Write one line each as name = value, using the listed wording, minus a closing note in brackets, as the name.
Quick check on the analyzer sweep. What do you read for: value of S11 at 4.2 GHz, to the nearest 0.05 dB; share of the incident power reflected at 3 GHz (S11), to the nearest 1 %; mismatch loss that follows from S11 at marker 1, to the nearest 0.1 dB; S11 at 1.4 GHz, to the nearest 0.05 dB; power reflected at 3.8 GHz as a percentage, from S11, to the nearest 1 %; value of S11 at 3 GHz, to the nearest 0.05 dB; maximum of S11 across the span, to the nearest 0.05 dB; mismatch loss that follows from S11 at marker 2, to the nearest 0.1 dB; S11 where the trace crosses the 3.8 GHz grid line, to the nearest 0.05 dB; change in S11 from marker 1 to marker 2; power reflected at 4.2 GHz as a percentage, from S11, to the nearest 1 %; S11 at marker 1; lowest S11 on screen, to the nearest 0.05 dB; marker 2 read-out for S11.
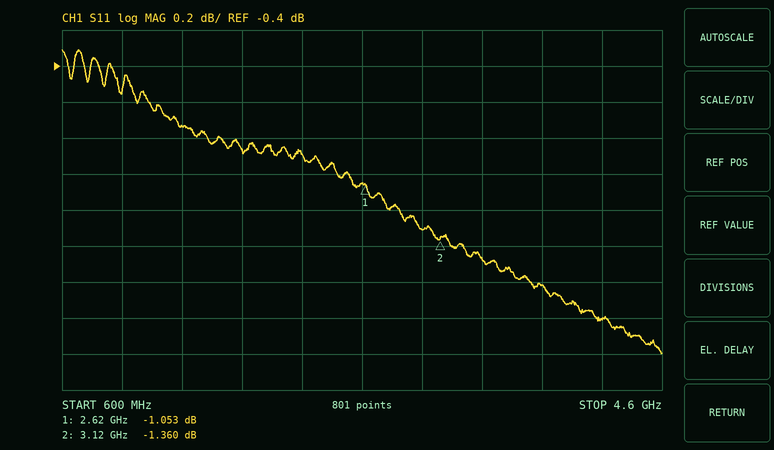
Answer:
value of S11 at 4.2 GHz, to the nearest 0.05 dB = -1.80 dB
share of the incident power reflected at 3 GHz (S11), to the nearest 1 % = 74 %
mismatch loss that follows from S11 at marker 1, to the nearest 0.1 dB = 6.7 dB
S11 at 1.4 GHz, to the nearest 0.05 dB = -0.75 dB
power reflected at 3.8 GHz as a percentage, from S11, to the nearest 1 % = 69 %
value of S11 at 3 GHz, to the nearest 0.05 dB = -1.30 dB
maximum of S11 across the span, to the nearest 0.05 dB = -0.30 dB
mismatch loss that follows from S11 at marker 2, to the nearest 0.1 dB = 5.7 dB
S11 where the trace crosses the 3.8 GHz grid line, to the nearest 0.05 dB = -1.60 dB
change in S11 from marker 1 to marker 2 = -0.307 dB
power reflected at 4.2 GHz as a percentage, from S11, to the nearest 1 % = 66 %
S11 at marker 1 = -1.053 dB
lowest S11 on screen, to the nearest 0.05 dB = -2.00 dB
marker 2 read-out for S11 = -1.360 dB
